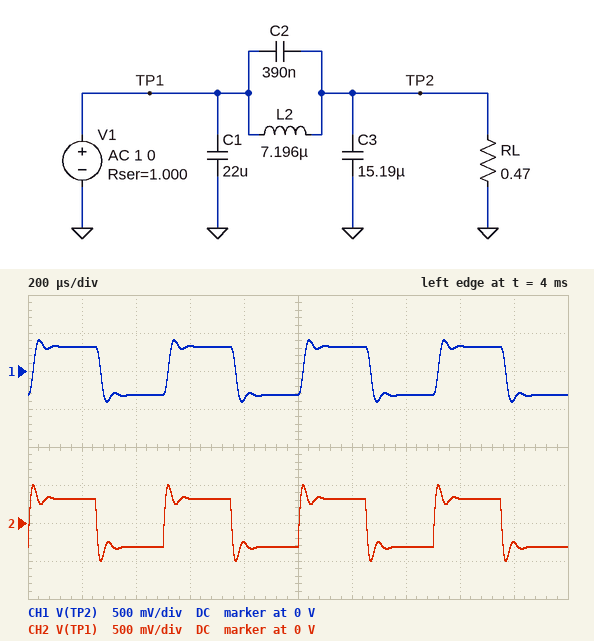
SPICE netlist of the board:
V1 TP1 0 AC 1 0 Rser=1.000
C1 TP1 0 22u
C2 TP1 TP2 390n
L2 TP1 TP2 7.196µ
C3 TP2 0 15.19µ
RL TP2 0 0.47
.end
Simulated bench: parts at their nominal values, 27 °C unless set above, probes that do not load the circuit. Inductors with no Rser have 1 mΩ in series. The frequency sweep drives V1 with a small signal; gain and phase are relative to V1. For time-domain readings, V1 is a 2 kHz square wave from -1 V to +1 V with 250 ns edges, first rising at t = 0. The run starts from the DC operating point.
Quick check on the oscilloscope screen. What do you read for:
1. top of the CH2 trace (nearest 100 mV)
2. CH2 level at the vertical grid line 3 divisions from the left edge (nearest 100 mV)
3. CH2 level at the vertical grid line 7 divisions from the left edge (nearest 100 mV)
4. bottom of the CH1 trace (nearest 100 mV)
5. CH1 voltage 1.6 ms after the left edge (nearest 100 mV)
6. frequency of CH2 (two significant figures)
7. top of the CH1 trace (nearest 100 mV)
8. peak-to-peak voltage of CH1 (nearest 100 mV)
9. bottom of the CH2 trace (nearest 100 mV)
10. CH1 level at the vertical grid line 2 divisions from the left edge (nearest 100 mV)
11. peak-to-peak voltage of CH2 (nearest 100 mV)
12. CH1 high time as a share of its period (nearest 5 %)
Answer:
500 mV
300 mV
-300 mV
-400 mV
300 mV
2.0 kHz
400 mV
800 mV
-500 mV
-300 mV
1.0 V
50 %
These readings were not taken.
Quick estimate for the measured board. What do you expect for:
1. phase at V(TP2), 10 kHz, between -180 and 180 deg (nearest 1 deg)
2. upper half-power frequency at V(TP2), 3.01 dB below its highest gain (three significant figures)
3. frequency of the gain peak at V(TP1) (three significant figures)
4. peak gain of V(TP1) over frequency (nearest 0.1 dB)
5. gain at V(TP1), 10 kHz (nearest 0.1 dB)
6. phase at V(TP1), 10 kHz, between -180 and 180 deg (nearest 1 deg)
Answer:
-64 deg
19.3 kHz
17.3 kHz
-5.9 dB
-8.6 dB
-4 deg
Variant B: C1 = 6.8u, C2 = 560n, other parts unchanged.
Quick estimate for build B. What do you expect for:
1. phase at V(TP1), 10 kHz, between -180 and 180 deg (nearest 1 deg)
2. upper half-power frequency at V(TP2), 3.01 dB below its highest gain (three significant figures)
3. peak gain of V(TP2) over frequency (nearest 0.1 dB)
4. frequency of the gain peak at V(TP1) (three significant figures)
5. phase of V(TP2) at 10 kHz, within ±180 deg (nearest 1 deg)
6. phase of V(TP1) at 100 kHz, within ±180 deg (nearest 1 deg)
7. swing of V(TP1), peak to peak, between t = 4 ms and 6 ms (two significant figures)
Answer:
16 deg
26.5 kHz
-9.9 dB
26.8 kHz
-44 deg
-77 deg
1.6 V
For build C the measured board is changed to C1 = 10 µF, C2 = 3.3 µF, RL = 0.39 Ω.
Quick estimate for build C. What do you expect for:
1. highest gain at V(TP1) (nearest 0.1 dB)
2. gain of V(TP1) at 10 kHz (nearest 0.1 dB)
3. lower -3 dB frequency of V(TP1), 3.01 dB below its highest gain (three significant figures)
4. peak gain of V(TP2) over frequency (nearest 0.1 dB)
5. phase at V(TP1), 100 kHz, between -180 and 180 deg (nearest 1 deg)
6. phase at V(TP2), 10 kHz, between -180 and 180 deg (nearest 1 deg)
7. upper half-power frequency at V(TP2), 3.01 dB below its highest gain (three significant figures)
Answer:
-1.9 dB
-7.9 dB
13.6 kHz
-10.6 dB
-82 deg
-48 deg
19.5 kHz
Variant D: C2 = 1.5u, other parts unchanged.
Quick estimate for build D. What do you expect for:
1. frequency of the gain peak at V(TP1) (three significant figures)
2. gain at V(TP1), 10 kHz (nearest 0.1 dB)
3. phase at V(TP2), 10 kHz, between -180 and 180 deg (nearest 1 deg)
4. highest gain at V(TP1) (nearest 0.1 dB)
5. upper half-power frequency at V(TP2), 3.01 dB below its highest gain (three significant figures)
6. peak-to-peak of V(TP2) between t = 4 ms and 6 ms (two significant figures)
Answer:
16.5 kHz
-8.4 dB
-65 deg
-5.6 dB
18.1 kHz
820 mV
